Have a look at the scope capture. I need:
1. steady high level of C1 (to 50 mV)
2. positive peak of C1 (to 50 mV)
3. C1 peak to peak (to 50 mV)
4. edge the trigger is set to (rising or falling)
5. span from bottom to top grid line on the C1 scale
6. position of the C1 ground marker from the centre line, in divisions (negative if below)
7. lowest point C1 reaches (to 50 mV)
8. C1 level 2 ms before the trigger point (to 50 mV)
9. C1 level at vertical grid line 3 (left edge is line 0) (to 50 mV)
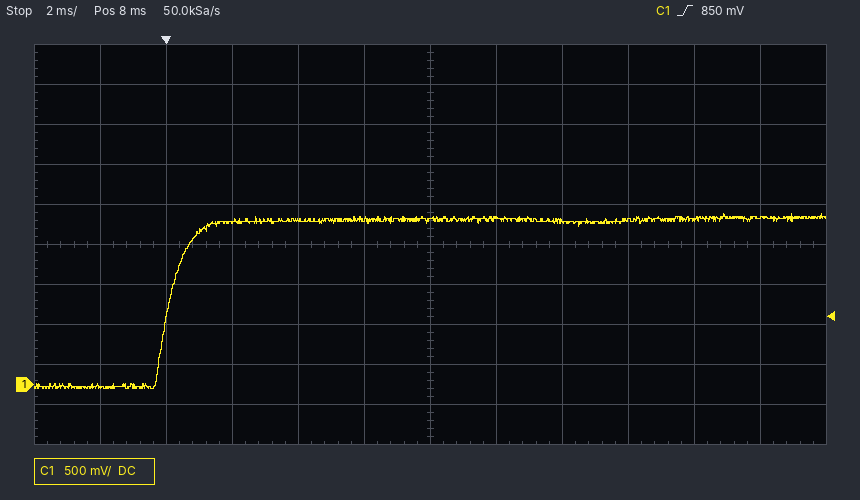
2.05 V
2.15 V
2.20 V
rising
5 V
-3.5 div
-50 mV
0 mV
2.05 V
